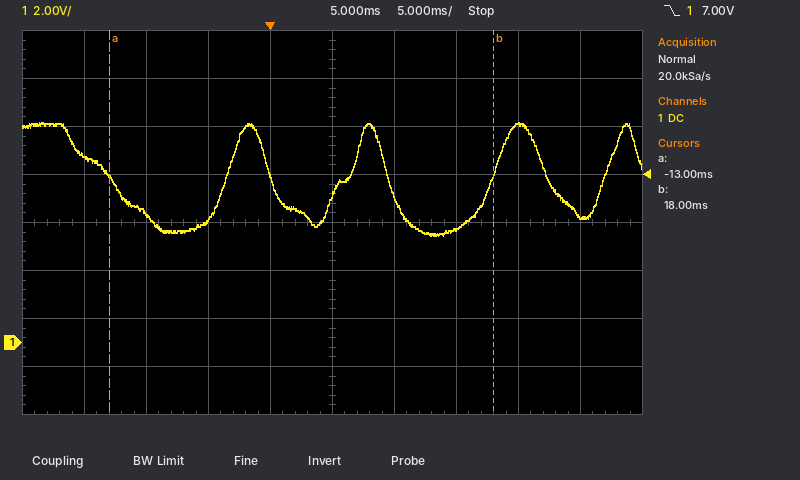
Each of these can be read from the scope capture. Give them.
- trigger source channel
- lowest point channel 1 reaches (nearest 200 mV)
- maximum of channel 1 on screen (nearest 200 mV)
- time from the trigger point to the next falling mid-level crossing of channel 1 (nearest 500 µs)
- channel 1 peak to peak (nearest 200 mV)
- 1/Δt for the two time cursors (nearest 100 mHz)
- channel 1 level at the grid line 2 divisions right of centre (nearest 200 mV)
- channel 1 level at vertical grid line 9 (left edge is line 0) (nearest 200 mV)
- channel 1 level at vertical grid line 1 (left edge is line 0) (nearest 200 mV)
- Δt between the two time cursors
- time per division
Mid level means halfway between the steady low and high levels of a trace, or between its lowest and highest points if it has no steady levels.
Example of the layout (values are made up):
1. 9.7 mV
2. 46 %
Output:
1. channel 1
2. 4.4 V
3. 9.2 V
4. 9.5 ms
5. 4.8 V
6. 32.3 Hz
7. 4.8 V
8. 5.2 V
9. 7.8 V
10. 31.0 ms
11. 5 ms
